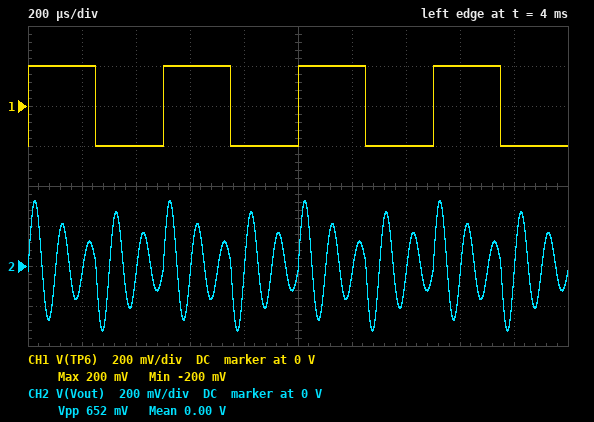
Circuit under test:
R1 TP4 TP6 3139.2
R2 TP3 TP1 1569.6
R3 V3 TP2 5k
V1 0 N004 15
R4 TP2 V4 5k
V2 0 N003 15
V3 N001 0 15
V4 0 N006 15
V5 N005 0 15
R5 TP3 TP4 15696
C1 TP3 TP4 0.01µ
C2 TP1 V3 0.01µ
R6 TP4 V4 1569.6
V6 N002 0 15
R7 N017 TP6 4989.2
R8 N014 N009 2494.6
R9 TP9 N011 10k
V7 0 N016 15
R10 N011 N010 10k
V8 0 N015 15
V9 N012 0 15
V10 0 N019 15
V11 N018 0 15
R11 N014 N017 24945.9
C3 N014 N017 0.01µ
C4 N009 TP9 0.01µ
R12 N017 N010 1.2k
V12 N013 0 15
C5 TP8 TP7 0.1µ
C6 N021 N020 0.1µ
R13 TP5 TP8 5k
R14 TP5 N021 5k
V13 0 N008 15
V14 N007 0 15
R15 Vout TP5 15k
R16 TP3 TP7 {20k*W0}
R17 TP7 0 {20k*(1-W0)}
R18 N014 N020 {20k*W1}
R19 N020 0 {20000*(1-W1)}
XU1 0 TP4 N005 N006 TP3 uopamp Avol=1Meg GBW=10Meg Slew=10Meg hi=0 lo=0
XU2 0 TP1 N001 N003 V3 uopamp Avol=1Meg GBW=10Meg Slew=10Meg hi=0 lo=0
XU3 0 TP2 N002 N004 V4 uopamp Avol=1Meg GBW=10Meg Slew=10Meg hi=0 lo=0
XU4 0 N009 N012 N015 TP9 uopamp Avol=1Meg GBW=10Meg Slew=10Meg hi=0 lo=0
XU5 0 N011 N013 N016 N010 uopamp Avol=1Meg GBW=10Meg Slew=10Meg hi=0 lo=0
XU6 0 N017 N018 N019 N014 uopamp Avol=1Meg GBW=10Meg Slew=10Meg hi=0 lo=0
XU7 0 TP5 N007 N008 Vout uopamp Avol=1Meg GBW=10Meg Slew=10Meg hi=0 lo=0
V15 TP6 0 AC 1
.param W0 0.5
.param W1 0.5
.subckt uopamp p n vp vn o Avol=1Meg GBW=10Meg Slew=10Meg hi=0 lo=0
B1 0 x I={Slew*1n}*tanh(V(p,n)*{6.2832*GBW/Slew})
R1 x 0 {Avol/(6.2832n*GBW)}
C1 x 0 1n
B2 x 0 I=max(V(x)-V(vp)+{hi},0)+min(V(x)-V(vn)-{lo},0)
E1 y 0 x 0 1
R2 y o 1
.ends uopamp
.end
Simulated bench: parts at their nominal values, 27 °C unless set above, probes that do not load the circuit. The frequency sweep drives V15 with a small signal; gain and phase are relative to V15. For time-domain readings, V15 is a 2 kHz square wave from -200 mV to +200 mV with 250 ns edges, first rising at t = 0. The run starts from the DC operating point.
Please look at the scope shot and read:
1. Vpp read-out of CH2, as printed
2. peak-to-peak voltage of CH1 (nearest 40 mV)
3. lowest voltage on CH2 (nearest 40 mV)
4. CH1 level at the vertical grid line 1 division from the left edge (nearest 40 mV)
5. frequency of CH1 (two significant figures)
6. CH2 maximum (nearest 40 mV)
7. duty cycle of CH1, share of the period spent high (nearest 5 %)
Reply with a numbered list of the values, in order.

1. 652 mV
2. 400 mV
3. -320 mV
4. 200 mV
5. 2.0 kHz
6. 320 mV
7. 50 %
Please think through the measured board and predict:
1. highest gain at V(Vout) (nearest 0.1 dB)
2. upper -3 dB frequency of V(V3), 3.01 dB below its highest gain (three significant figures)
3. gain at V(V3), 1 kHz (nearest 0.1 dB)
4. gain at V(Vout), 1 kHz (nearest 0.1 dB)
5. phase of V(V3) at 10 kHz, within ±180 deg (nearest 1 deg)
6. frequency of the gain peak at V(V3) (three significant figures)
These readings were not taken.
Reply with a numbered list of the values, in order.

1. 14.0 dB
2. 10.6 kHz
3. -5.9 dB
4. -23.7 dB
5. -75 deg
6. 10.1 kHz
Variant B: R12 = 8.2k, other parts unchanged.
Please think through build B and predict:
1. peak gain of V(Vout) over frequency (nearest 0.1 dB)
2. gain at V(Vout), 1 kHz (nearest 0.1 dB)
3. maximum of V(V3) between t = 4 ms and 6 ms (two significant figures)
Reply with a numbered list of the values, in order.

1. 11.9 dB
2. -12.2 dB
3. 420 mV
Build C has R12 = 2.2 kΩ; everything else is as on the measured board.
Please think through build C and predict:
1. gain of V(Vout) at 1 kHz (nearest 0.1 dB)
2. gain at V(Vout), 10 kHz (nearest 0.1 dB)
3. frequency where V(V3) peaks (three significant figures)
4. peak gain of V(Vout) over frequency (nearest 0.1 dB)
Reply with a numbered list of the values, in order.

1. -21.0 dB
2. 11.5 dB
3. 10.1 kHz
4. 12.0 dB
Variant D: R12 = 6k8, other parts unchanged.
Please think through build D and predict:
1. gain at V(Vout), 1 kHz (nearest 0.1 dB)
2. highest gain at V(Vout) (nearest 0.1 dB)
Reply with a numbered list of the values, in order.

1. -13.7 dB
2. 11.9 dB
